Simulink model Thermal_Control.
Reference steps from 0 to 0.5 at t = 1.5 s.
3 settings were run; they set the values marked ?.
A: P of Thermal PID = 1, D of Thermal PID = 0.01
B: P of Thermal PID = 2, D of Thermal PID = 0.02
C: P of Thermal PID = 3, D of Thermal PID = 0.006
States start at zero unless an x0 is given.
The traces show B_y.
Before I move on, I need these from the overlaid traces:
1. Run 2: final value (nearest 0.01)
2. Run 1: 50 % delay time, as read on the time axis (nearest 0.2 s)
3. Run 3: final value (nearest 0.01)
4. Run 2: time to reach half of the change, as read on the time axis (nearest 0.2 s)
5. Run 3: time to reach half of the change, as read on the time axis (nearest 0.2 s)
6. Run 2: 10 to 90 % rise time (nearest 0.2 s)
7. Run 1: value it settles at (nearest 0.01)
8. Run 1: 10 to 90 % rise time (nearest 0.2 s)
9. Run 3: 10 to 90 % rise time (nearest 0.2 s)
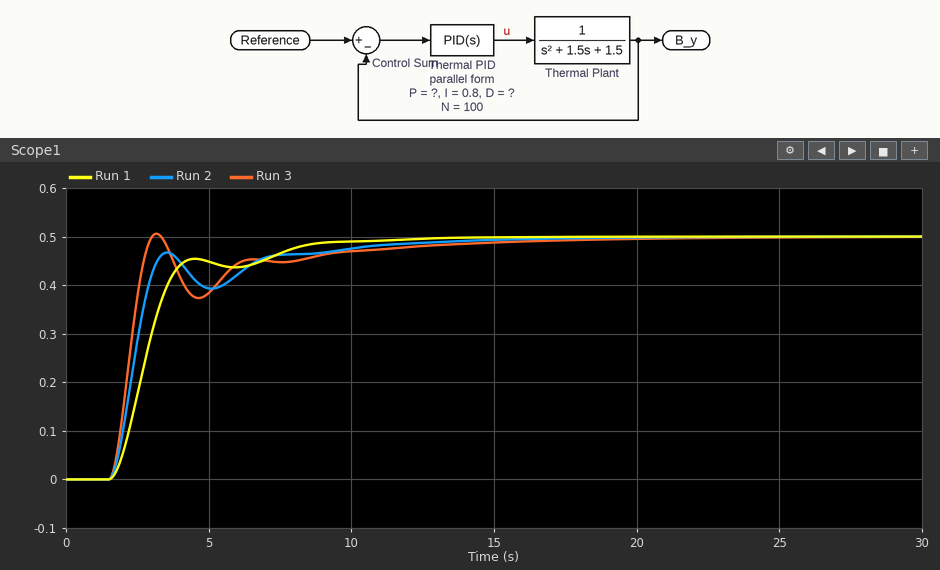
0.50
2.8 s
0.50
2.4 s
2.2 s
1.4 s
0.50
2.2 s
1.0 s
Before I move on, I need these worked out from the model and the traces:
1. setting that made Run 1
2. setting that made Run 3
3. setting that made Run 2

A
C
B
